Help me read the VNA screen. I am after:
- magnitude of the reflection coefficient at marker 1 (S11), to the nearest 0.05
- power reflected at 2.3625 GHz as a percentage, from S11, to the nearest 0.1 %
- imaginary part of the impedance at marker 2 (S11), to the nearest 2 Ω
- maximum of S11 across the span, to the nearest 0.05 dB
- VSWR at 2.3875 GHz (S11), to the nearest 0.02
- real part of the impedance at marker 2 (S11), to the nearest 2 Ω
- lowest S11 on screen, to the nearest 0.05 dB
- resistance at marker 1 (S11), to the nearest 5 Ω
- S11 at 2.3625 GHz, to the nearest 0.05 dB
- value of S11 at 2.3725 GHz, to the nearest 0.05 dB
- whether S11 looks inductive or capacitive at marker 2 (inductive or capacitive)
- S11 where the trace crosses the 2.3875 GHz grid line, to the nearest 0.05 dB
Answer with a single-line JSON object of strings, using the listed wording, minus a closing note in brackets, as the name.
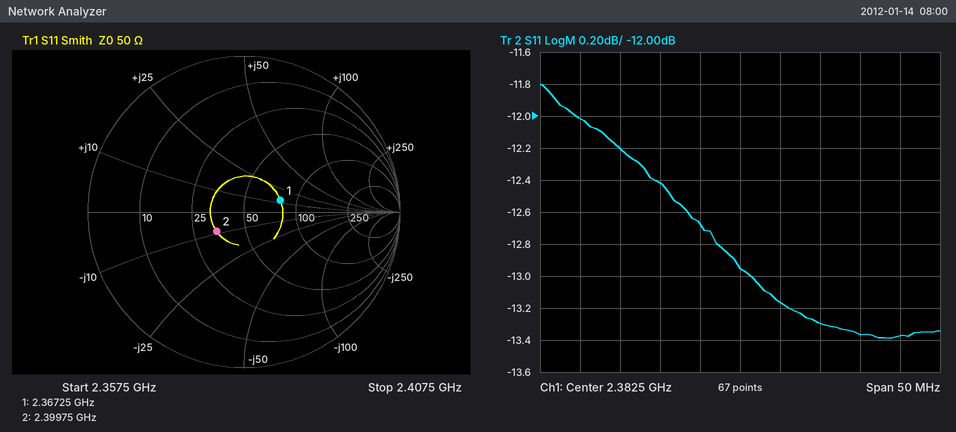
{"magnitude of the reflection coefficient at marker 1 (S11), to the nearest 0.05": "0.25", "power reflected at 2.3625 GHz as a percentage, from S11, to the nearest 0.1 %": "6.3 %", "imaginary part of the impedance at marker 2 (S11), to the nearest 2 Ω": "-8 Ω", "maximum of S11 across the span, to the nearest 0.05 dB": "-11.80 dB", "VSWR at 2.3875 GHz (S11), to the nearest 0.02": "1.56", "real part of the impedance at marker 2 (S11), to the nearest 2 Ω": "34 Ω", "lowest S11 on screen, to the nearest 0.05 dB": "-13.40 dB", "resistance at marker 1 (S11), to the nearest 5 Ω": "80 Ω", "S11 at 2.3625 GHz, to the nearest 0.05 dB": "-12.00 dB", "value of S11 at 2.3725 GHz, to the nearest 0.05 dB": "-12.40 dB", "whether S11 looks inductive or capacitive at marker 2": "capacitive", "S11 where the trace crosses the 2.3875 GHz grid line, to the nearest 0.05 dB": "-13.15 dB"}
